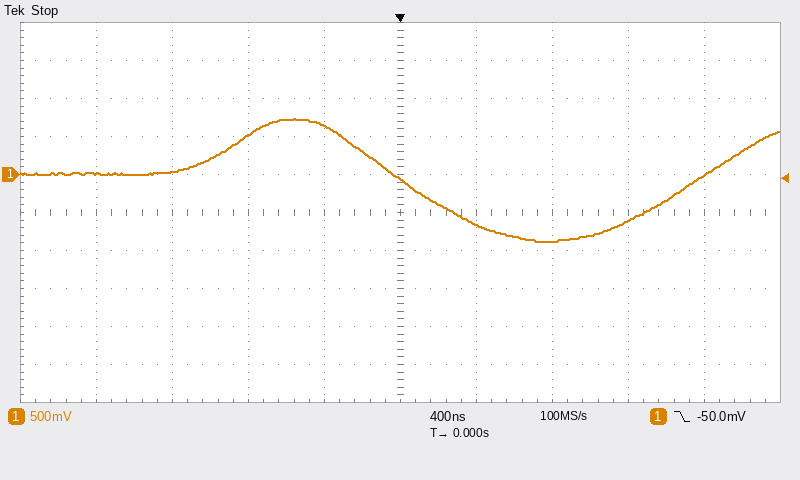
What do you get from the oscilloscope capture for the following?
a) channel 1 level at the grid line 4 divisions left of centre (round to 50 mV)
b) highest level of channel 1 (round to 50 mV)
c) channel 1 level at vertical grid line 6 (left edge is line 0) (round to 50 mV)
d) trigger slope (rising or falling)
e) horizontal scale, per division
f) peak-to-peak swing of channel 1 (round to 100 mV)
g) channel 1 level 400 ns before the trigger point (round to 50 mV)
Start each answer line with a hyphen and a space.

- 0 mV
- 750 mV
- -650 mV
- falling
- 400 ns
- 1.60 V
- 650 mV
